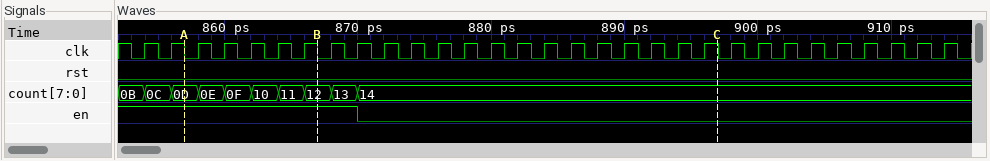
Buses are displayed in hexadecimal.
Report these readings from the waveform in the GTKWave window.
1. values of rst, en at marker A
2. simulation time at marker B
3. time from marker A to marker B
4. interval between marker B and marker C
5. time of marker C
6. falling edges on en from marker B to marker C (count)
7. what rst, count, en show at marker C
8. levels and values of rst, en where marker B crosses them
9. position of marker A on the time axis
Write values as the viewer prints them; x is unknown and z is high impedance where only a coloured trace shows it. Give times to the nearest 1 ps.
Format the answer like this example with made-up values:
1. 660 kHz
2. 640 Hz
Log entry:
1. rst=0, en=1
2. 867 ps
3. 10 ps
4. 30 ps
5. 897 ps
6. 1
7. rst=0, count=14, en=0
8. rst=0, en=1
9. 857 ps
